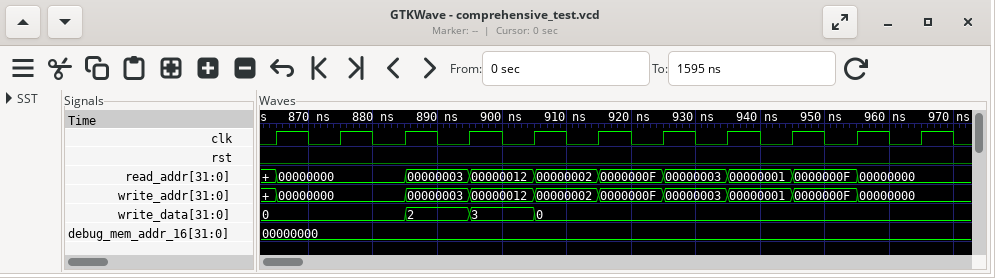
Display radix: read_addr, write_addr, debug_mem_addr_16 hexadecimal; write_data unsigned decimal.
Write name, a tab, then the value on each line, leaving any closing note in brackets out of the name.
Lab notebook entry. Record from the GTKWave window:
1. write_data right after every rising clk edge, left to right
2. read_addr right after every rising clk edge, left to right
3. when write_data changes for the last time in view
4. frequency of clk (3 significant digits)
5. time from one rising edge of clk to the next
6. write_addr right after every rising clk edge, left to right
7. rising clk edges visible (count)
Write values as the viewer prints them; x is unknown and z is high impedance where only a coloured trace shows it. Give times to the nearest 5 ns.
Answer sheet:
write_data right after every rising clk edge, left to right	0, 0, 2, 3, 0, 0, 0, 0, 0, 0, 0
read_addr right after every rising clk edge, left to right	00000000, 00000000, 00000003, 00000012, 00000002, 0000000F, 00000003, 00000001, 0000000F, 00000000, 00000000
when write_data changes for the last time in view	905 ns
frequency of clk	100 MHz
time from one rising edge of clk to the next	10 ns
write_addr right after every rising clk edge, left to right	00000000, 00000000, 00000003, 00000012, 00000002, 0000000F, 00000003, 00000001, 0000000F, 00000000, 00000000
rising clk edges visible	11
